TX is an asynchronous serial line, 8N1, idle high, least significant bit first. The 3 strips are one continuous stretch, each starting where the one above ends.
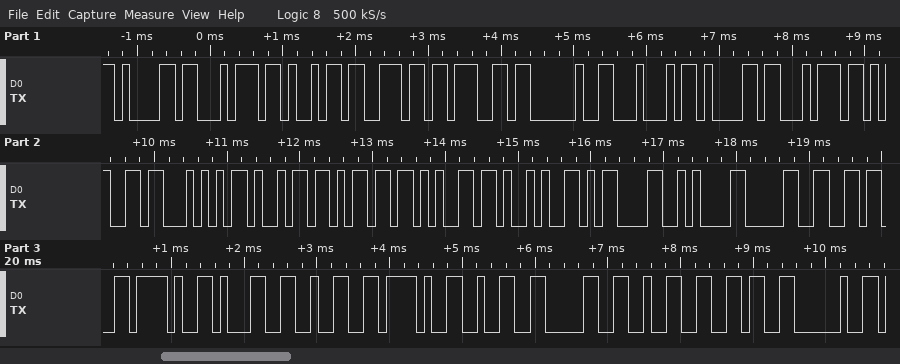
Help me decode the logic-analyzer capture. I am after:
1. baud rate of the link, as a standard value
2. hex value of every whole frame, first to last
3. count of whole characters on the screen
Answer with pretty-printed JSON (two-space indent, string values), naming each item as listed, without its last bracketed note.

{
  "baud rate of the link, as a standard value": "9600 baud",
  "hex value of every whole frame, first to last": "0x61 0x74 0x69 0x6E 0x67 0x20 0x44 0x61 0x74 0x65 0x54 0x69 0x6D 0x65 0x29 0x0D 0x0A 0x30 0x36 0x2F 0x31 0x32 0x2F 0x32 0x30 0x32 0x36 0x20",
  "count of whole characters on the screen": "28"
}
